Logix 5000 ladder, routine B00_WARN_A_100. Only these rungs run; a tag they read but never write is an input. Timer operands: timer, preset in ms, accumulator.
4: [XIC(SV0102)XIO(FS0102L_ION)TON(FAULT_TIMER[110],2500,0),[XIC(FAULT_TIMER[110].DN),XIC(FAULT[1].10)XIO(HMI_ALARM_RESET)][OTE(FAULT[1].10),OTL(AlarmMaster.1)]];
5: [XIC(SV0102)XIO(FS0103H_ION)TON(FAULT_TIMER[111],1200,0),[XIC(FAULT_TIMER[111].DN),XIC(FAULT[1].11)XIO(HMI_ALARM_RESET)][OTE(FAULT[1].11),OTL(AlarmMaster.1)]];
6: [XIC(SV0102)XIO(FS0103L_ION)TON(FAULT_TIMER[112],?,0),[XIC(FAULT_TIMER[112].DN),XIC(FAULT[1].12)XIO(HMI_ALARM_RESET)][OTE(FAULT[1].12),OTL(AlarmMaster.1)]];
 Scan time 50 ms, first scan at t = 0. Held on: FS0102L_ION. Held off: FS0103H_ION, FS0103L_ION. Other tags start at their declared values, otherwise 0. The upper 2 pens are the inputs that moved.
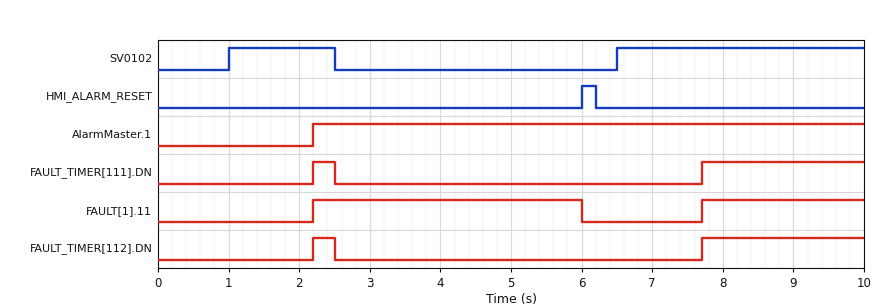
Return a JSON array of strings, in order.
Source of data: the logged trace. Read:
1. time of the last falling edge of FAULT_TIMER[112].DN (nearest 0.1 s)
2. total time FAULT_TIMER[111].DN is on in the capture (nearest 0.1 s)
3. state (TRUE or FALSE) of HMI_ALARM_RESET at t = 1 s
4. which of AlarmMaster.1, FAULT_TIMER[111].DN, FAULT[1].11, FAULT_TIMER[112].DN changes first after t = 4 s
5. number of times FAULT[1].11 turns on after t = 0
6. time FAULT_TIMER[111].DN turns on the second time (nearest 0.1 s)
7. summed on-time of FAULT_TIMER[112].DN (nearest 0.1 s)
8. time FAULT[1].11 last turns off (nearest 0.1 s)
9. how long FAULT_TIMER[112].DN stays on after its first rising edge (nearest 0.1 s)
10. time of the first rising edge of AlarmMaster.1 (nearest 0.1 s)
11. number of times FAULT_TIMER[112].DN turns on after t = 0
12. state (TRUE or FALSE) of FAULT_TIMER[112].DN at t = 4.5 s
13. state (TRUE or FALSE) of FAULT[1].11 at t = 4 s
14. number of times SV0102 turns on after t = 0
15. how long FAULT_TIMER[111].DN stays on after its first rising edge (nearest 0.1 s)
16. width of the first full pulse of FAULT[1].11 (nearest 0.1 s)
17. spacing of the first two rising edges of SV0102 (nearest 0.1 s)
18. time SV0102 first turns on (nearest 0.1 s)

["2.5 s", "2.6 s", "FALSE", "FAULT[1].11", "2", "7.7 s", "2.6 s", "6.0 s", "0.3 s", "2.2 s", "2", "FALSE", "TRUE", "2", "0.3 s", "3.8 s", "5.5 s", "1.0 s"]
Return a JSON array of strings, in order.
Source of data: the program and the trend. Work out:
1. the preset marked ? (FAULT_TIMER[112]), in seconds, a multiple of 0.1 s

["1.2 s"]
